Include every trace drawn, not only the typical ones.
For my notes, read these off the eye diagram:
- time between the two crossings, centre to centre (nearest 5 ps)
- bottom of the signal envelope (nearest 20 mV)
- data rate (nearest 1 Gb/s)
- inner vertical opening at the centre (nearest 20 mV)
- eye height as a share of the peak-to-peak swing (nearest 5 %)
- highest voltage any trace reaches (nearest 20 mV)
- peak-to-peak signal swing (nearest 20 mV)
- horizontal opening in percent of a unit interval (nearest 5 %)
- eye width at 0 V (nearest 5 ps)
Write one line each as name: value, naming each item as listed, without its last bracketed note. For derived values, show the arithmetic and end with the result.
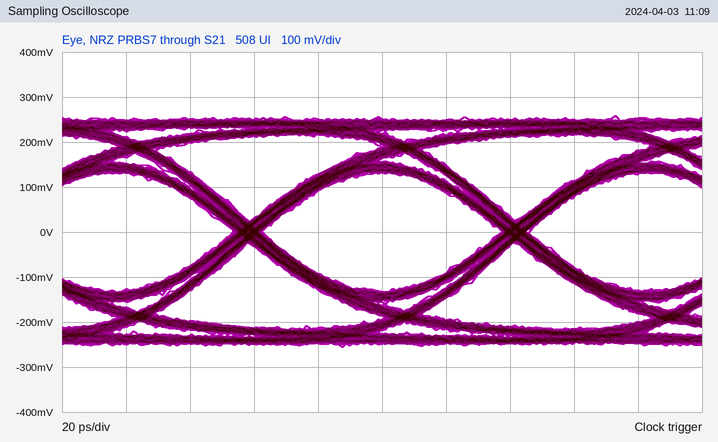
time between the two crossings, centre to centre: 85 ps
bottom of the signal envelope: -260 mV
data rate: 12 Gb/s
inner vertical opening at the centre: 260 mV
eye height as a share of the peak-to-peak swing: 260 mV / 520 mV ≈ 50 %
highest voltage any trace reaches: 260 mV
peak-to-peak signal swing: 520 mV
horizontal opening in percent of a unit interval: 75 ps / 85 ps ≈ 88.2 %, so 90 % to the nearest 5 %
eye width at 0 V: 75 ps
